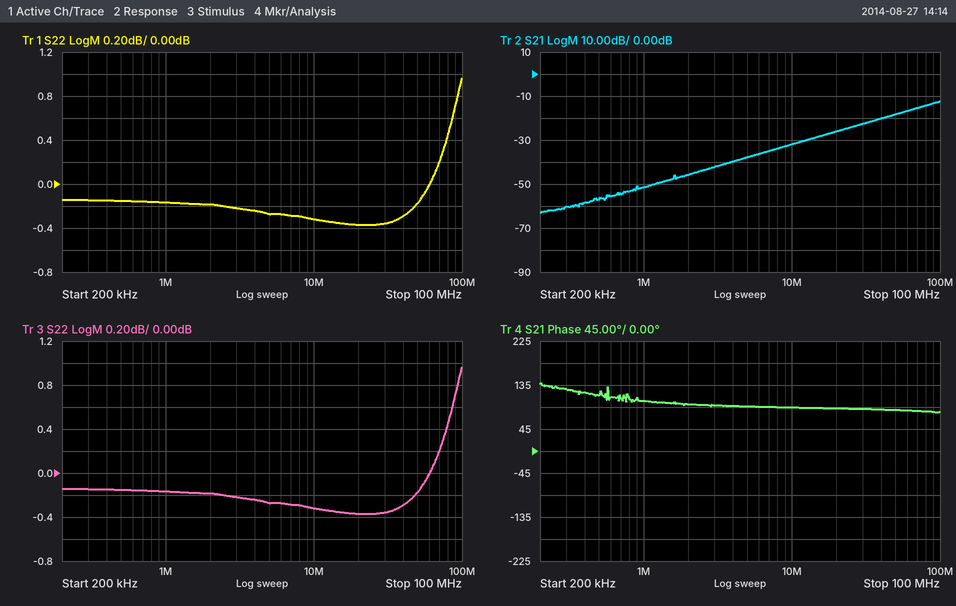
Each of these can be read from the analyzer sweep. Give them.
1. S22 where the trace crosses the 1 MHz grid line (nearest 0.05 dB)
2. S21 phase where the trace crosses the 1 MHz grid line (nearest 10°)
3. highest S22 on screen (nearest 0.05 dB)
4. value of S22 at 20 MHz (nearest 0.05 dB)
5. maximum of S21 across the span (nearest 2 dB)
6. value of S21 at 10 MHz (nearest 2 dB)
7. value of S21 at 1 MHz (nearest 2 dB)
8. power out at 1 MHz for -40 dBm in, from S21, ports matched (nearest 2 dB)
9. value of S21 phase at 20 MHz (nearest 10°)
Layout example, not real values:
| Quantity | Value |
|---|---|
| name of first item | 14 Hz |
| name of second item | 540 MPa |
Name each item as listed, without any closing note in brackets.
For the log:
| Quantity | Value |
|---|---|
| S22 where the trace crosses the 1 MHz grid line | -0.15 dB |
| S21 phase where the trace crosses the 1 MHz grid line | 100° |
| highest S22 on screen | 0.95 dB |
| value of S22 at 20 MHz | -0.35 dB |
| maximum of S21 across the span | -12 dB |
| value of S21 at 10 MHz | -32 dB |
| value of S21 at 1 MHz | -52 dB |
| power out at 1 MHz for -40 dBm in, from S21, ports matched | -92 dBm |
| value of S21 phase at 20 MHz | 90° |
